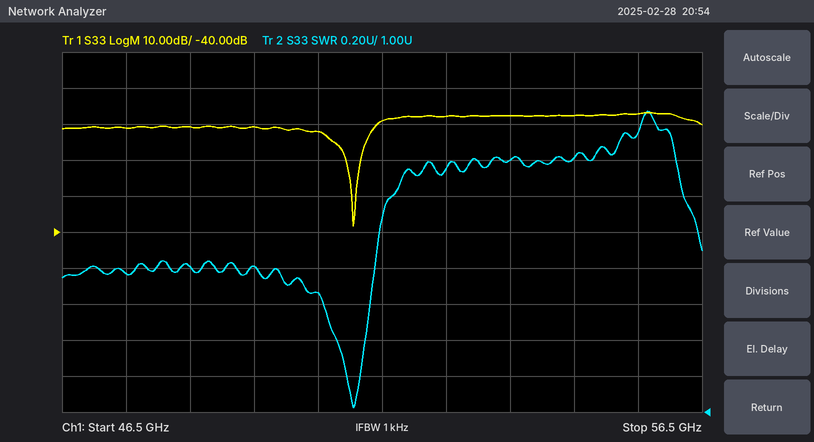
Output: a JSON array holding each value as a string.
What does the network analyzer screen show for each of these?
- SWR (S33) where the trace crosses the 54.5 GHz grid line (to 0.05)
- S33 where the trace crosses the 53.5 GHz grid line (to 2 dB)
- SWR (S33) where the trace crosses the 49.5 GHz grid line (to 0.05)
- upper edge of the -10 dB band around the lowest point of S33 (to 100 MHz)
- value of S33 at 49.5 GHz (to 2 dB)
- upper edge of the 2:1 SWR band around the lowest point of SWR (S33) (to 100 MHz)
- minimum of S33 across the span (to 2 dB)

["2.40", "-8 dB", "1.80", "51.4 GHz", "-10 dB", "51.5 GHz", "-38 dB"]
